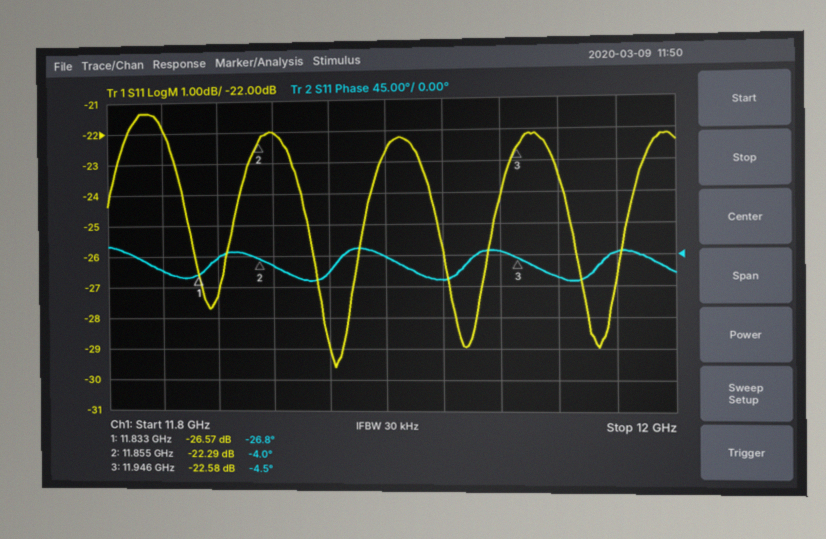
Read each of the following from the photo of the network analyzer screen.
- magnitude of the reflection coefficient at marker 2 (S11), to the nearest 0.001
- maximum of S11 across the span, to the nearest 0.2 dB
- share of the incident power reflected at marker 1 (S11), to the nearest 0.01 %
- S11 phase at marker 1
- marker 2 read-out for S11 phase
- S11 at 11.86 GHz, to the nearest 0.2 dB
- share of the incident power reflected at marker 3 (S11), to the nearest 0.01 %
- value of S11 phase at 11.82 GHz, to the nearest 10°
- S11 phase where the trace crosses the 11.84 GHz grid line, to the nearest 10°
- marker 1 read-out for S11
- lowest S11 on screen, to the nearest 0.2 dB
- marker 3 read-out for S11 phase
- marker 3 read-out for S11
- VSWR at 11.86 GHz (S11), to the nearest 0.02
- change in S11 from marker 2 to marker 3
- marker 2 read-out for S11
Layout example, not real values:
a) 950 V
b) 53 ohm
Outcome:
a) 0.077
b) -21.4 dB
c) 0.22 %
d) -26.8°
e) -4.0°
f) -22.0 dB
g) 0.55 %
h) -20°
i) 0°
j) -26.57 dB
k) -29.6 dB
l) -4.5°
m) -22.58 dB
n) 1.18
o) -0.29 dB
p) -22.29 dB
